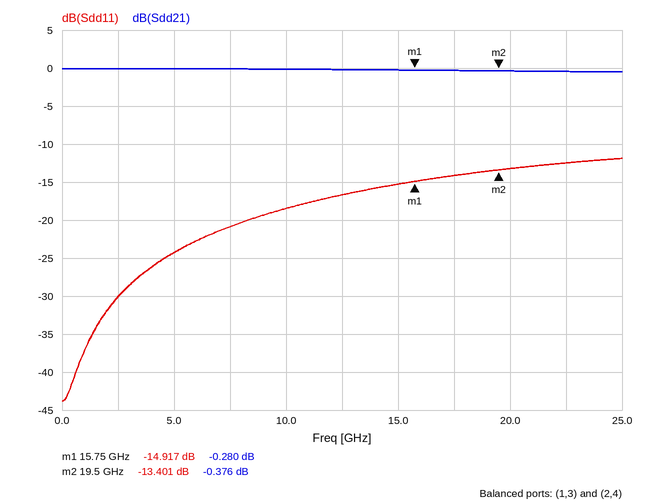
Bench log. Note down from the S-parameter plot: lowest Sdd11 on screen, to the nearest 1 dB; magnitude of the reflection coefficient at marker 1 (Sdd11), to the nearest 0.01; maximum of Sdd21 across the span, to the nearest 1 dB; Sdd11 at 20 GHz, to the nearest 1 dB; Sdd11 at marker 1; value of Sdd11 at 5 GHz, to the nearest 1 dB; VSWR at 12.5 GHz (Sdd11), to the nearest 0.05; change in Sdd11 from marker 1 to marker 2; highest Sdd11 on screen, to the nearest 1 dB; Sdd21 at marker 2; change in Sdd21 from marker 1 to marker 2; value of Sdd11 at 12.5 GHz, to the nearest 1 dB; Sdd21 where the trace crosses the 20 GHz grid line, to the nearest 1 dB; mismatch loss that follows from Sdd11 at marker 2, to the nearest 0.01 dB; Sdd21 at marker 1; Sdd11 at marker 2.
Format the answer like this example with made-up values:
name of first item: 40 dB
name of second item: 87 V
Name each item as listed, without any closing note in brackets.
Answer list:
lowest Sdd11 on screen, to the nearest 1 dB: -44 dB
magnitude of the reflection coefficient at marker 1 (Sdd11), to the nearest 0.01: 0.18
maximum of Sdd21 across the span, to the nearest 1 dB: 0 dB
Sdd11 at 20 GHz, to the nearest 1 dB: -13 dB
Sdd11 at marker 1: -14.917 dB
value of Sdd11 at 5 GHz, to the nearest 1 dB: -24 dB
VSWR at 12.5 GHz (Sdd11), to the nearest 0.05: 1.35
change in Sdd11 from marker 1 to marker 2: 1.516 dB
highest Sdd11 on screen, to the nearest 1 dB: -12 dB
Sdd21 at marker 2: -0.376 dB
change in Sdd21 from marker 1 to marker 2: -0.096 dB
value of Sdd11 at 12.5 GHz, to the nearest 1 dB: -17 dB
Sdd21 where the trace crosses the 20 GHz grid line, to the nearest 1 dB: 0 dB
mismatch loss that follows from Sdd11 at marker 2, to the nearest 0.01 dB: 0.20 dB
Sdd21 at marker 1: -0.280 dB
Sdd11 at marker 2: -13.401 dB
